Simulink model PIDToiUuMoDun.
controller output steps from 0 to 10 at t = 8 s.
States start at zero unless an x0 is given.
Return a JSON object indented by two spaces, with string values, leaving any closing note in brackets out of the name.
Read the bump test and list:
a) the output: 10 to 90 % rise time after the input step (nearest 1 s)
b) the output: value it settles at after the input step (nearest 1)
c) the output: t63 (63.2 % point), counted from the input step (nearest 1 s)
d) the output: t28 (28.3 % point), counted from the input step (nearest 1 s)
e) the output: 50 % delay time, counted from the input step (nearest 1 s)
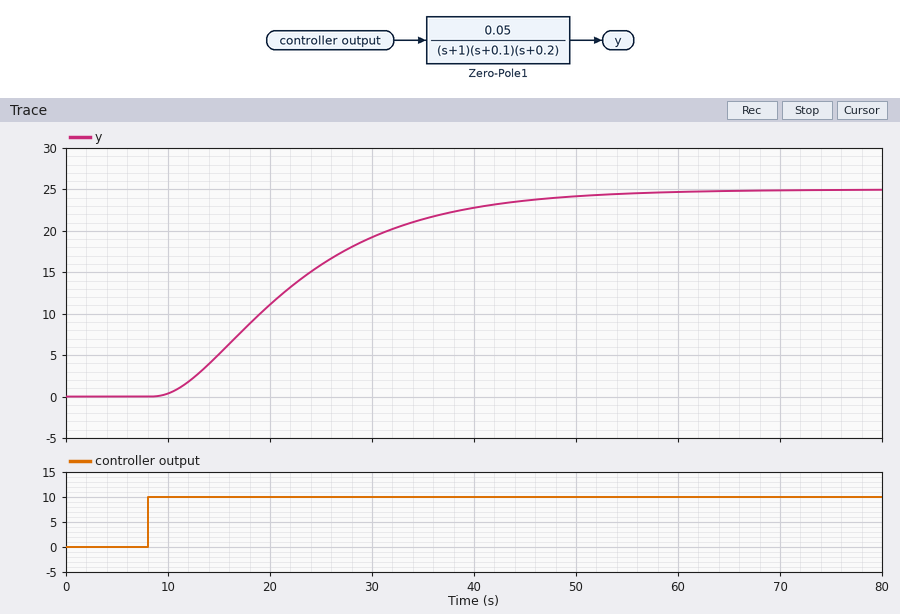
{
  "the output: 10 to 90 % rise time after the input step": "26 s",
  "the output: value it settles at after the input step": "25",
  "the output: t63 (63.2 % point), counted from the input step": "17 s",
  "the output: t28 (28.3 % point), counted from the input step": "9 s",
  "the output: 50 % delay time, counted from the input step": "13 s"
}
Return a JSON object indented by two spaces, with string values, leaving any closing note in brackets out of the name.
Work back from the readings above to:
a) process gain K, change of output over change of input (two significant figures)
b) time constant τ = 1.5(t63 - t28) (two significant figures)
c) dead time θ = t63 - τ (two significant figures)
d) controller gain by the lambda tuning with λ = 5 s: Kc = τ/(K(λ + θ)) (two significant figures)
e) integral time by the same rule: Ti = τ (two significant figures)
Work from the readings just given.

{
  "process gain K, change of output over change of input": "2.5",
  "time constant τ = 1.5(t63 - t28)": "12 s",
  "dead time θ = t63 - τ": "5.0 s",
  "controller gain by the lambda tuning with λ = 5 s: Kc = τ/(K(λ + θ))": "0.48",
  "integral time by the same rule: Ti = τ": "12 s"
}
